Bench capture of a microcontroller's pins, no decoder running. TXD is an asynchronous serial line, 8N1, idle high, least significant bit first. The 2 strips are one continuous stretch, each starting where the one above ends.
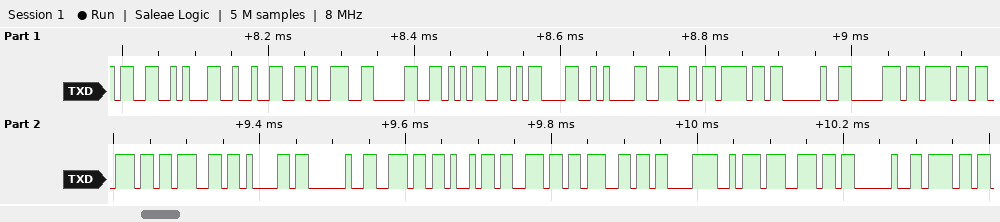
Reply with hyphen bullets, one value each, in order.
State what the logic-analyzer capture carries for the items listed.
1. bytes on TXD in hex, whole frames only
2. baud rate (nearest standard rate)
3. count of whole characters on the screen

- 33 31 32 39 30 35 0D 0A 4E 6F 20 70 6F 6E 67 61 20 6E 69 6E 67 C3 BA 6E 20 6F
- 115200 baud
- 26
